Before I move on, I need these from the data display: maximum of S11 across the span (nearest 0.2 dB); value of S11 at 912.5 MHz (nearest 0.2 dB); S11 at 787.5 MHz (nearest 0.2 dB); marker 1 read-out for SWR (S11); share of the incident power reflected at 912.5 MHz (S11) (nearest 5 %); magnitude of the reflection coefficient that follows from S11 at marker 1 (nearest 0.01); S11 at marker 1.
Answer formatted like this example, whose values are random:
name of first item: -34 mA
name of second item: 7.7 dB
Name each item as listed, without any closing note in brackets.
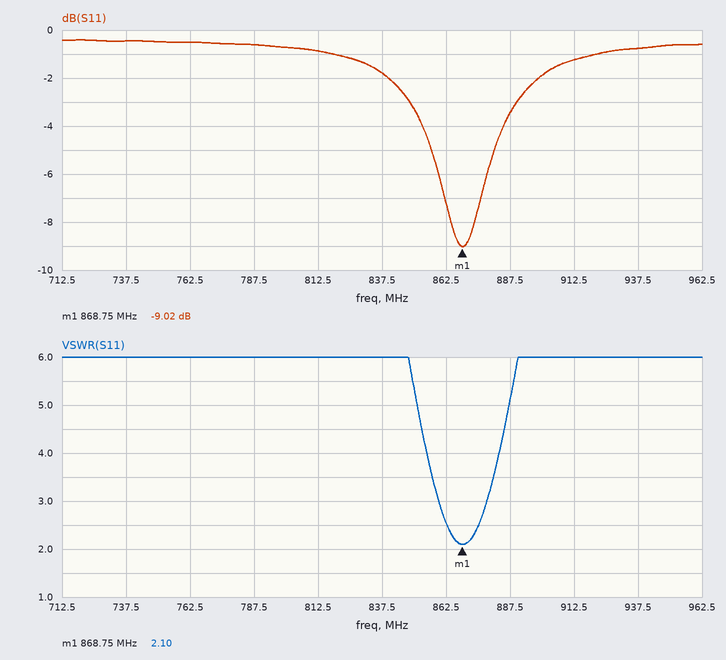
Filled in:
maximum of S11 across the span: -0.4 dB
value of S11 at 912.5 MHz: -1.2 dB
S11 at 787.5 MHz: -0.6 dB
marker 1 read-out for SWR: 2.10
share of the incident power reflected at 912.5 MHz (S11): 75 %
magnitude of the reflection coefficient that follows from S11 at marker 1: 0.35
S11 at marker 1: -9.02 dB
